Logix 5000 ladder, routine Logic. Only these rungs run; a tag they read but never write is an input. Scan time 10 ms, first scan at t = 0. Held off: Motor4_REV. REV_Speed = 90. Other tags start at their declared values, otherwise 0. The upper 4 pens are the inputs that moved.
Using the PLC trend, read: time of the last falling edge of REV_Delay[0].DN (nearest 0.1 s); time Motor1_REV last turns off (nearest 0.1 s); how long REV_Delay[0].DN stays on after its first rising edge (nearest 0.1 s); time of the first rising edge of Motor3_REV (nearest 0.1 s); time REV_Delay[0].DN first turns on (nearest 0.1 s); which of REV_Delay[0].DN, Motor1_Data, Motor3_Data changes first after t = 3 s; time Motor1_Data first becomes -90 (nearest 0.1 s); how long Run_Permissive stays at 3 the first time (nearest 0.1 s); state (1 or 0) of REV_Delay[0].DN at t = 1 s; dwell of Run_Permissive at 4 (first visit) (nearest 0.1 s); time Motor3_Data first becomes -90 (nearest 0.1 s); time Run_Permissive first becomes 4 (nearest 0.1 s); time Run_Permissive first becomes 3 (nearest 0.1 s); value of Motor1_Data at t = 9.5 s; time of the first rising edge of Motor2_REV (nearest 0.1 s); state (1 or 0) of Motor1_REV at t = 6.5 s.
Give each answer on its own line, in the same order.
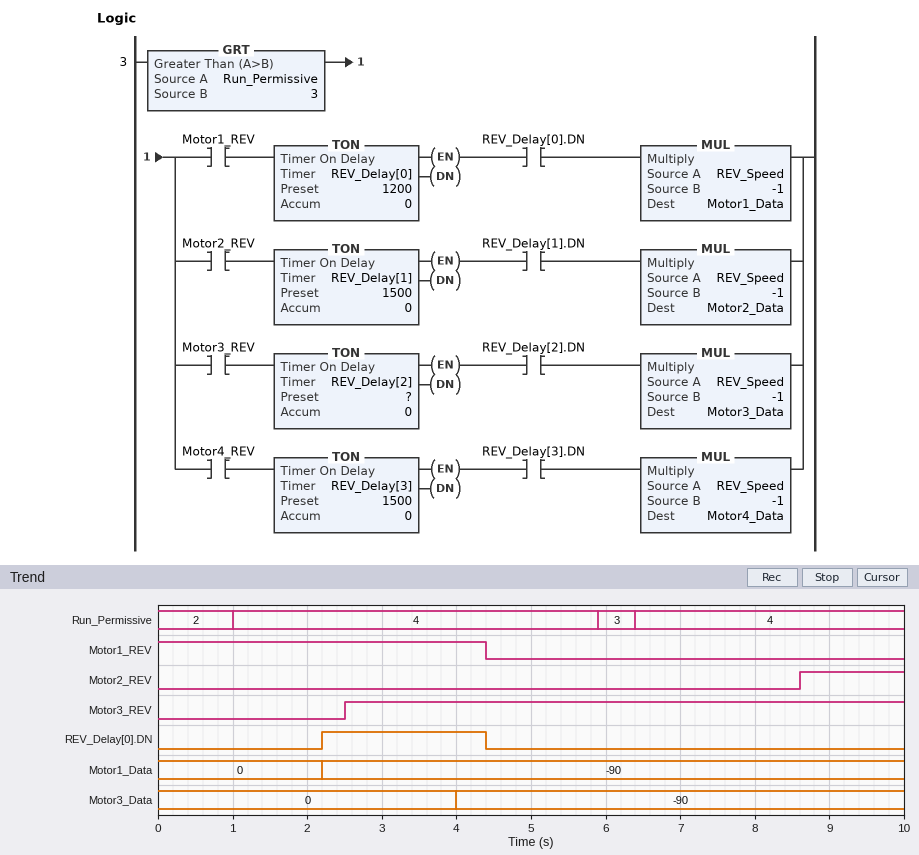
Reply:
4.4 s
4.4 s
2.2 s
2.5 s
2.2 s
Motor3_Data
2.2 s
0.5 s
0
4.9 s
4.0 s
1.0 s
5.9 s
-90
8.6 s
0
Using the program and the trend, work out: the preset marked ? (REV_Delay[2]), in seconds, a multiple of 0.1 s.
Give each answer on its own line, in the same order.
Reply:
1.5 s
